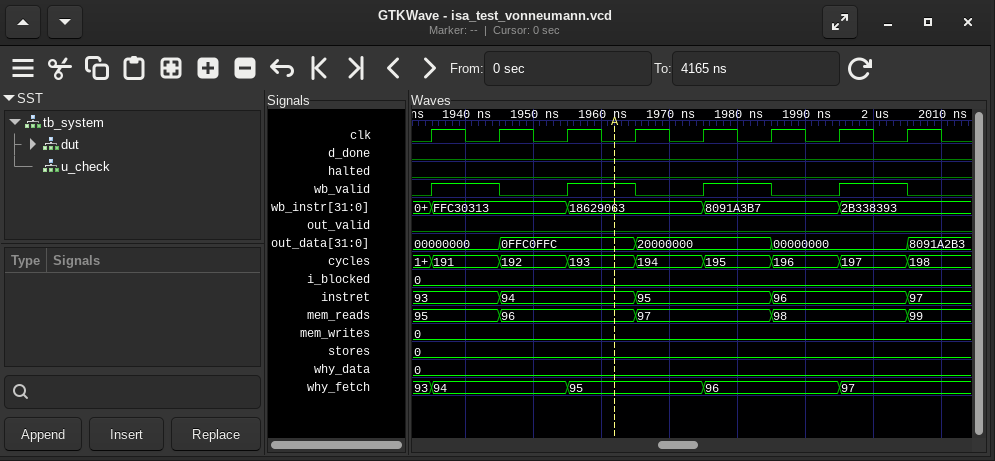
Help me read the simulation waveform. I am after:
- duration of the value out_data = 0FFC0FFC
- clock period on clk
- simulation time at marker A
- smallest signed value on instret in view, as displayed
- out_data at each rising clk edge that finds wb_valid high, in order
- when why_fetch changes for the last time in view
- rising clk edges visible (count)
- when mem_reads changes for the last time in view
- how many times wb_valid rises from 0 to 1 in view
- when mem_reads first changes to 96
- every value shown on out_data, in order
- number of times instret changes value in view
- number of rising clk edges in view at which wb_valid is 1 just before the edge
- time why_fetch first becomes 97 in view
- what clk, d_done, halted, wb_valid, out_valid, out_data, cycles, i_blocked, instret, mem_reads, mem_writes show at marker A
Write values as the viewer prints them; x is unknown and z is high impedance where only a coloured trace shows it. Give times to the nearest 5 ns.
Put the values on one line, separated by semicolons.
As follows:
20 ns; 10 ns; 1960 ns; 93; 00000000, 0FFC0FFC, 20000000, 00000000; 1995 ns; 8; 2005 ns; 4; 1945 ns; 00000000, 0FFC0FFC, 20000000, 00000000, 8091A2B3; 4; 4; 1995 ns; clk=0, d_done=0, halted=0, wb_valid=1, out_valid=0, out_data=0FFC0FFC, cycles=193, i_blocked=0, instret=94, mem_reads=96, mem_writes=0
